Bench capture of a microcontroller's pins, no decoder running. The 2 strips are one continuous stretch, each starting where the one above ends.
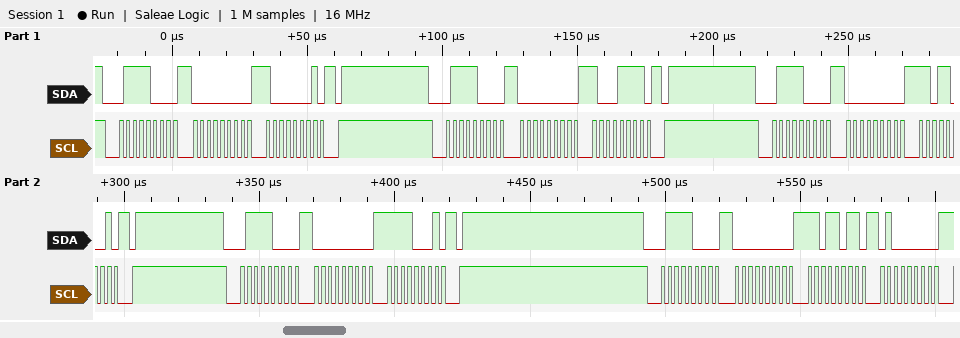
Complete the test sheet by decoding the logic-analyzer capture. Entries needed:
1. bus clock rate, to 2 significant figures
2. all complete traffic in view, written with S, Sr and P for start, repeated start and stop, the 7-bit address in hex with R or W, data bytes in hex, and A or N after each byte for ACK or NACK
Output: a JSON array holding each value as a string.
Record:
["400 kHz", "S 3CW A 00 A 81 A P S 3CW A 00 A 8F A P S 3CW A 00 A D9 A P S 3CW A 00 A F1 A P S 3CW A 00 A DB A 40 A"]
